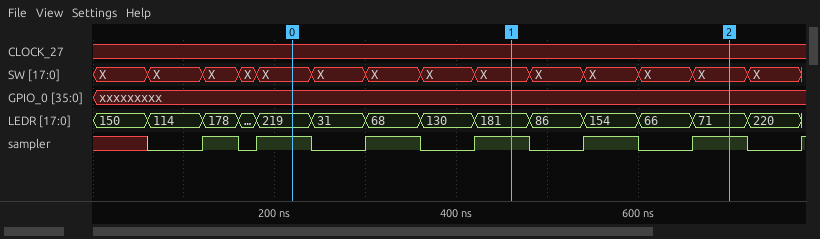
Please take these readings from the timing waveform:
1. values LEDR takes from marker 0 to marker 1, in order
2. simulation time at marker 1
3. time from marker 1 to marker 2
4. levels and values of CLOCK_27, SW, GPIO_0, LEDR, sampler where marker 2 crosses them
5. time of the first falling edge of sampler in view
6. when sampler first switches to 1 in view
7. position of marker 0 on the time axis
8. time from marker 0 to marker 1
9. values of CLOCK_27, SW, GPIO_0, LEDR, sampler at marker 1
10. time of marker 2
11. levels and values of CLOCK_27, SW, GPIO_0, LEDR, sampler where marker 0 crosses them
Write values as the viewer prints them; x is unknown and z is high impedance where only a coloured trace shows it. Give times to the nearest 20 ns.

219, 31, 68, 130, 181
460 ns
240 ns
CLOCK_27=x, SW=X, GPIO_0=xxxxxxxxx, LEDR=71, sampler=1
160 ns
120 ns
220 ns
240 ns
CLOCK_27=x, SW=X, GPIO_0=xxxxxxxxx, LEDR=181, sampler=1
700 ns
CLOCK_27=x, SW=X, GPIO_0=xxxxxxxxx, LEDR=219, sampler=1
